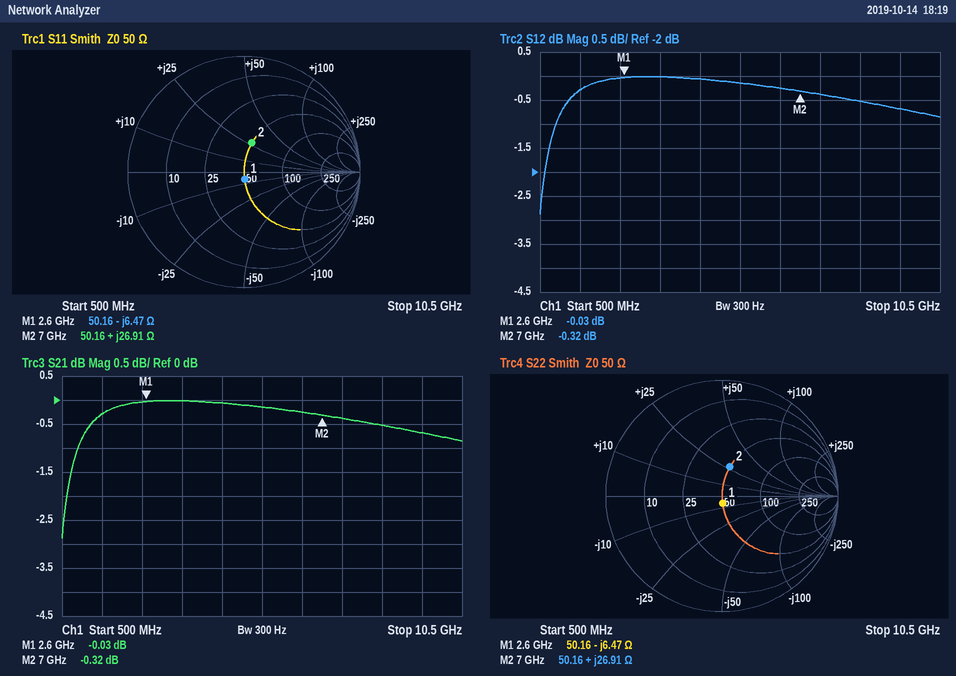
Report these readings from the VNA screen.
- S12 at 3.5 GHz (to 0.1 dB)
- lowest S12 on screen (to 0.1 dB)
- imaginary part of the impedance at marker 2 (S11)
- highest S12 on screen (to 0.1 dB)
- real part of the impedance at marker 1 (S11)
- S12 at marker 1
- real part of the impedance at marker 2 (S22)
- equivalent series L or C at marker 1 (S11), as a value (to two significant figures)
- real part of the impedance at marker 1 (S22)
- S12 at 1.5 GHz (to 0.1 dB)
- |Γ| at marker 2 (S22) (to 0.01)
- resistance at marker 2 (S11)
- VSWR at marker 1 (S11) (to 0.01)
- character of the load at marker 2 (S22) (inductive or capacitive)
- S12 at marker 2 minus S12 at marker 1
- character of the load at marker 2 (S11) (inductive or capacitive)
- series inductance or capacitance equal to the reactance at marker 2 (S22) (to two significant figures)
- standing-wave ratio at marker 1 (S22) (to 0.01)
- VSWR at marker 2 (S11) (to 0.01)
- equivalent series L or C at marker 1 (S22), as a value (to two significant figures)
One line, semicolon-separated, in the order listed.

0.0 dB; -2.9 dB; +26.91 Ω; 0.0 dB; 50.16 Ω; -0.03 dB; 50.16 Ω; 9.5 pF; 50.16 Ω; -0.3 dB; 0.26; 50.16 Ω; 1.14; inductive; -0.29 dB; inductive; 610 pH; 1.14; 1.70; 9.5 pF
